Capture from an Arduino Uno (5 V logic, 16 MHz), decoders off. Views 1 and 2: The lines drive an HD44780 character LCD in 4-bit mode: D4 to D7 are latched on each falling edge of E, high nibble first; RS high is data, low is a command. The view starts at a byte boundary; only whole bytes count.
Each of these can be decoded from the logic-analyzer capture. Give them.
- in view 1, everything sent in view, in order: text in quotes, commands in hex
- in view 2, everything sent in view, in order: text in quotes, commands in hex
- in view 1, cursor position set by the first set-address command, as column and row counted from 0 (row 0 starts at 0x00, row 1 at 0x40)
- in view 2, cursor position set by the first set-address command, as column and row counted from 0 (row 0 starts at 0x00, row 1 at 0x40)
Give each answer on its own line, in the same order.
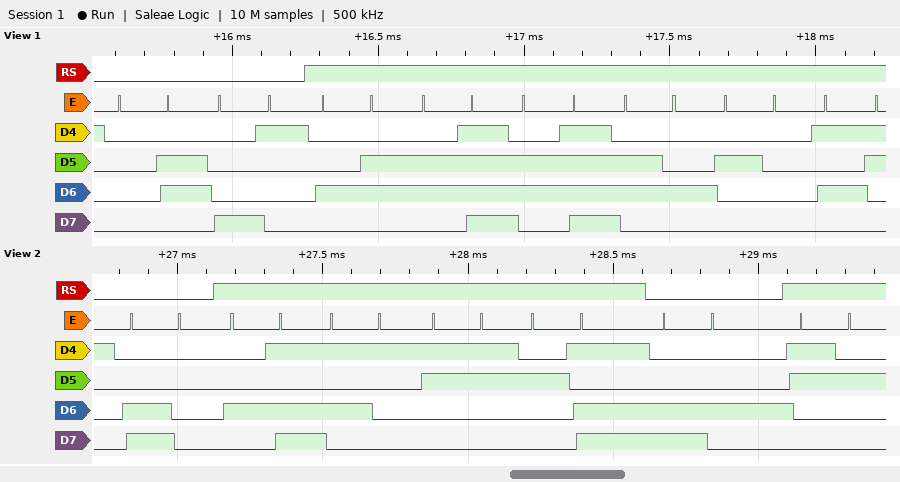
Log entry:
0x06 0x81 "Food S"
0xC0 "MQ3-" 0xC4 "2"
column 1, row 0
column 0, row 1
